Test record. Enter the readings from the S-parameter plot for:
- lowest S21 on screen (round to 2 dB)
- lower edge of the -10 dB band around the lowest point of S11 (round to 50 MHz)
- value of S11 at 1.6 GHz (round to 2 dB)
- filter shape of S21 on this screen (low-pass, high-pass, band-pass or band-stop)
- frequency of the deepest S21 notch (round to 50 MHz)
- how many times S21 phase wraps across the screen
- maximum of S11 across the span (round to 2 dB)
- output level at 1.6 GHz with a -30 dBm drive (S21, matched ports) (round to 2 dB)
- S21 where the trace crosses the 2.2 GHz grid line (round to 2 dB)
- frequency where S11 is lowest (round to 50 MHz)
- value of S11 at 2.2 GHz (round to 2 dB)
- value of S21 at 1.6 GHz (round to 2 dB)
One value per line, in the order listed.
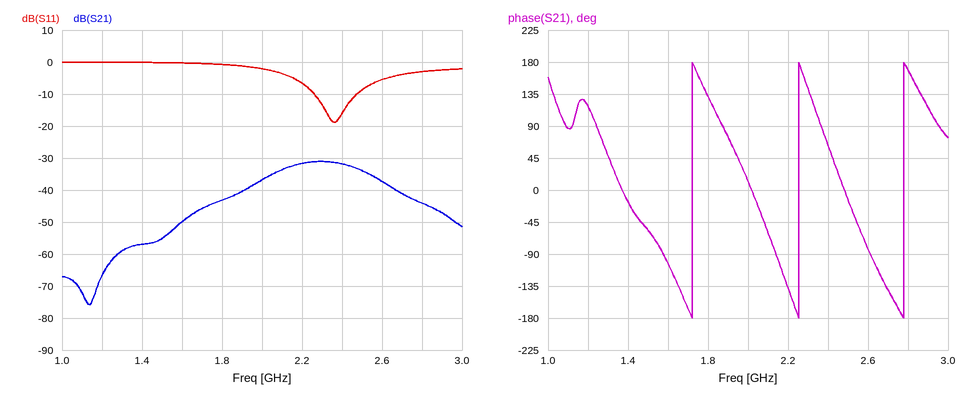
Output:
-76 dB
2.25 GHz
0 dB
band-pass
1.15 GHz
3
0 dB
-80 dBm
-32 dB
2.35 GHz
-6 dB
-50 dB
